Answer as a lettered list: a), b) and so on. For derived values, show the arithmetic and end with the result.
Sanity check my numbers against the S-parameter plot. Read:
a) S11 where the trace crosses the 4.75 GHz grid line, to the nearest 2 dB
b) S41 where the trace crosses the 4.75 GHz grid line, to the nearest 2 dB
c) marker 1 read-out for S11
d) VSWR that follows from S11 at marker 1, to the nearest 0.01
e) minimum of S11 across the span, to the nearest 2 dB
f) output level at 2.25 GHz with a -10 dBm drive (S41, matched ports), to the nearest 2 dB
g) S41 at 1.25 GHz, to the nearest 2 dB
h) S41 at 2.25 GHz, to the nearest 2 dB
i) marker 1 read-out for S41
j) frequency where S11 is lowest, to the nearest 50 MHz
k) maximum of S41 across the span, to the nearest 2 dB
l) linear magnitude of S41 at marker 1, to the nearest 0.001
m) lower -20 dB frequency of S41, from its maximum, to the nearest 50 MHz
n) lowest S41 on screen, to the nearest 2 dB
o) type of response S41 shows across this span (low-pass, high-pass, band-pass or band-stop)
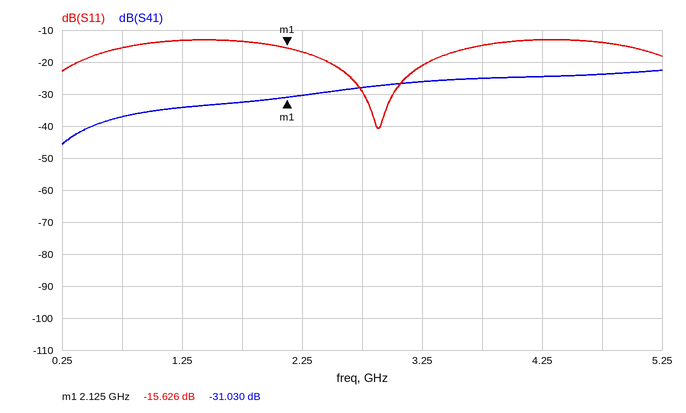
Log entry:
a) -14 dB
b) -24 dB
c) -15.626 dB
d) (1 + 0.1655)/(1 − 0.1655) ≈ 1.40
e) -40 dB
f) -10 dBm + (-30 dB) = -40 dBm
g) -34 dB
h) -30 dB
i) -31.030 dB
j) 2.90 GHz
k) -22 dB
l) 10^(-31.03/20) ≈ 0.028
m) 350 MHz
n) -46 dB
o) high-pass
